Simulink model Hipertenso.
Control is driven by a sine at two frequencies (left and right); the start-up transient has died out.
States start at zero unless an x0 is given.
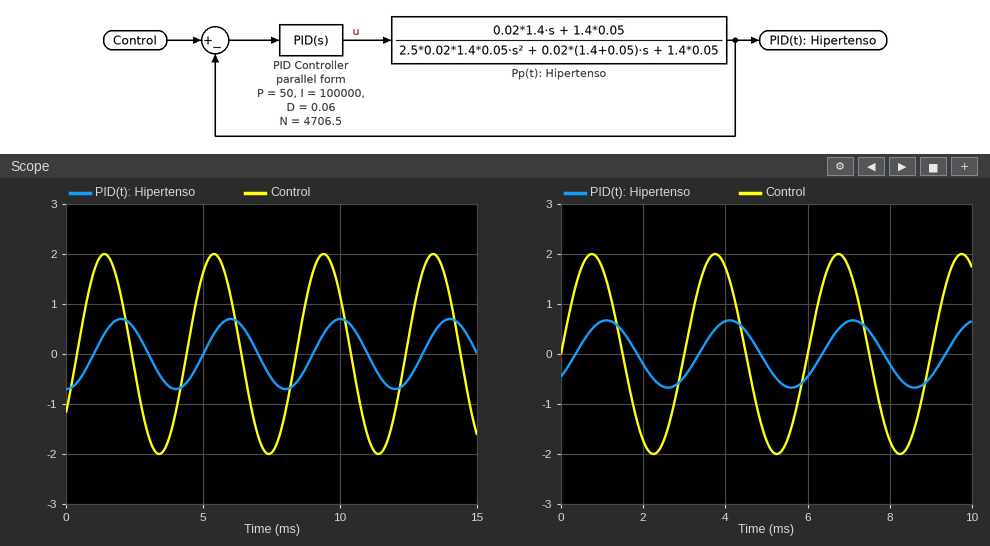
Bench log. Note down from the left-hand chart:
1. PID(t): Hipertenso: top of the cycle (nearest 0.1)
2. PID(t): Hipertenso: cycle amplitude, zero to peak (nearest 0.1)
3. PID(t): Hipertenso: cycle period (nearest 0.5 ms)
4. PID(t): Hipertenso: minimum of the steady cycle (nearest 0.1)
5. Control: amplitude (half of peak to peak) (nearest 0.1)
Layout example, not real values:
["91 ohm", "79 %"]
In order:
["0.7", "0.7", "4.0 ms", "-0.7", "2.0"]
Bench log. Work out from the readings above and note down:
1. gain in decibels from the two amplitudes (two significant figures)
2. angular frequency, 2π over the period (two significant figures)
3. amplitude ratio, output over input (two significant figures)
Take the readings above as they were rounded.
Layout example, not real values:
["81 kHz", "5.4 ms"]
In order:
["-9.1 dB", "1.6 rad/ms", "0.35"]
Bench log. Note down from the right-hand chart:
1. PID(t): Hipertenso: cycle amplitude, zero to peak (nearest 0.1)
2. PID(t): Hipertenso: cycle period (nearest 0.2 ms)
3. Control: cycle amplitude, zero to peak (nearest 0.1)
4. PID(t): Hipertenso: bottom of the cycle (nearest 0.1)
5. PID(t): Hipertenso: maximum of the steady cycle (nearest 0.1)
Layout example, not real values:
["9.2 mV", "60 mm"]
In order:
["0.7", "3.0 ms", "2.0", "-0.7", "0.7"]
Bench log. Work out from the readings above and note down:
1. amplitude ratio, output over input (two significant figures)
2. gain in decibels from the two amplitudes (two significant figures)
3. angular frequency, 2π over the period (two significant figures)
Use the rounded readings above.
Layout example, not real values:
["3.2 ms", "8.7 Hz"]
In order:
["0.35", "-9.1 dB", "2.1 rad/ms"]
